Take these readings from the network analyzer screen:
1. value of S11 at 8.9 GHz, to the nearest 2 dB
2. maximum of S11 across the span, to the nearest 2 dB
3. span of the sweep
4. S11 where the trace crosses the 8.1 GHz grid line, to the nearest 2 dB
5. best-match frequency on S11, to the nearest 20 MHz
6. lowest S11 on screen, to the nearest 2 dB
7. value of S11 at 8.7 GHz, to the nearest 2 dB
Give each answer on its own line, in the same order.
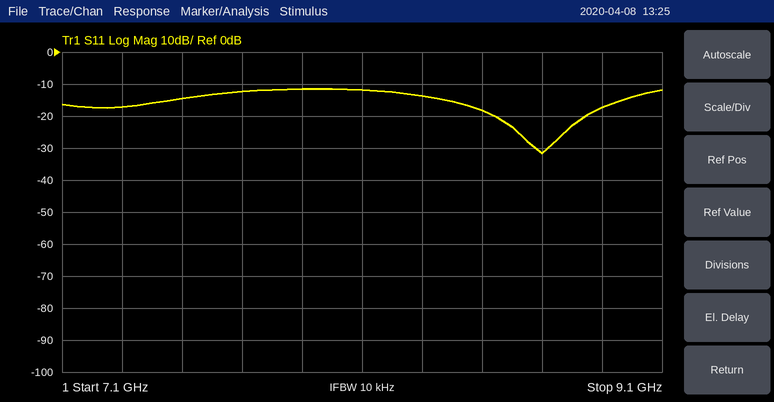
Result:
-18 dB
-12 dB
2 GHz
-12 dB
8.70 GHz
-32 dB
-32 dB
